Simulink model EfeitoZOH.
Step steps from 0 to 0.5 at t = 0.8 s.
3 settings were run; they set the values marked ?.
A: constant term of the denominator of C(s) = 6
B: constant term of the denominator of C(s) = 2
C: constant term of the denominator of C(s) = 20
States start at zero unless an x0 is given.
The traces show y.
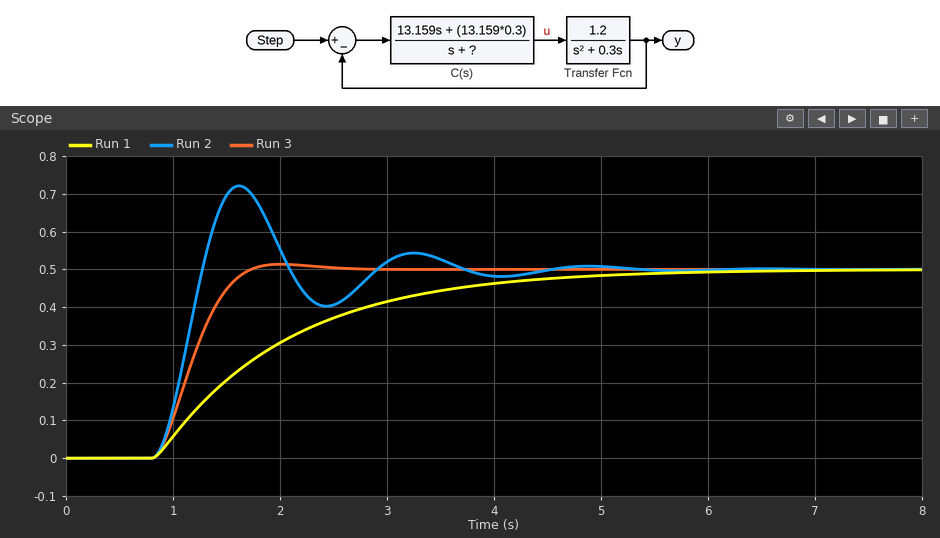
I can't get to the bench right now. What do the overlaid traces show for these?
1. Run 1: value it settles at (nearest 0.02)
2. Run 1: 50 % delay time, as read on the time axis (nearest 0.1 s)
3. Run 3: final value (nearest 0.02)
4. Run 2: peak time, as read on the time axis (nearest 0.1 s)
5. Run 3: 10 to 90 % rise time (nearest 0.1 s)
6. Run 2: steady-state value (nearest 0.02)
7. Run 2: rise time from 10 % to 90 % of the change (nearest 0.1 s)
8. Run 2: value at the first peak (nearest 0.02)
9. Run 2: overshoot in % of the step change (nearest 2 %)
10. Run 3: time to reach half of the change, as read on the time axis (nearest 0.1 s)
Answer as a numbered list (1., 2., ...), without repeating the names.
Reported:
1. 0.50
2. 1.7 s
3. 0.50
4. 1.6 s
5. 0.6 s
6. 0.50
7. 0.3 s
8. 0.72
9. 44 %
10. 1.2 s
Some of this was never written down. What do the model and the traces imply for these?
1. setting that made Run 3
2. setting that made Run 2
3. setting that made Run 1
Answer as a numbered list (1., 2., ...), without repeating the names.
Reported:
1. A
2. B
3. C
